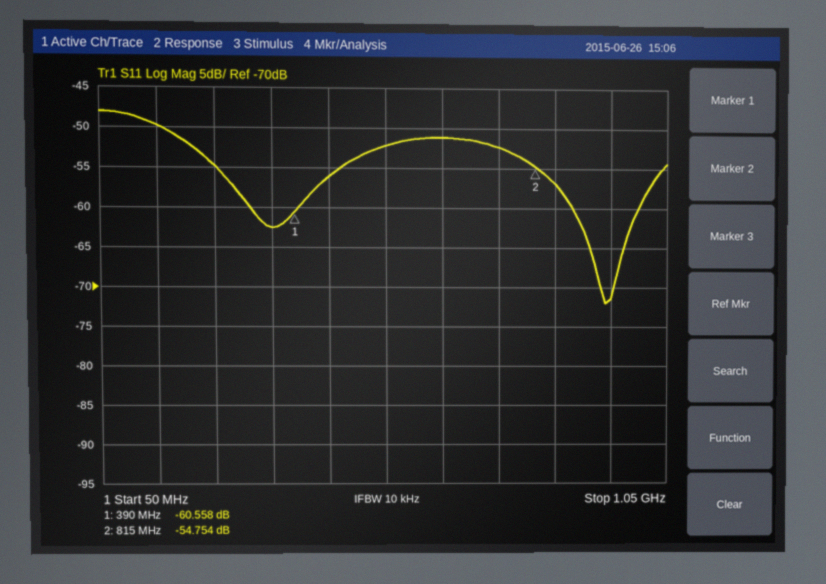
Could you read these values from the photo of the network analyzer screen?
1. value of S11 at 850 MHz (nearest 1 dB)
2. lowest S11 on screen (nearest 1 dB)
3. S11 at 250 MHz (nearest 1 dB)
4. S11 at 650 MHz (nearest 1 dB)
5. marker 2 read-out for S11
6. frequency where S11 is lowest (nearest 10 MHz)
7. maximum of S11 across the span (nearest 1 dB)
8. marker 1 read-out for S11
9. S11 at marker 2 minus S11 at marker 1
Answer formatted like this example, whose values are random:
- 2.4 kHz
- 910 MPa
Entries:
- -57 dB
- -72 dB
- -55 dB
- -51 dB
- -54.754 dB
- 940 MHz
- -48 dB
- -60.558 dB
- 5.804 dB
